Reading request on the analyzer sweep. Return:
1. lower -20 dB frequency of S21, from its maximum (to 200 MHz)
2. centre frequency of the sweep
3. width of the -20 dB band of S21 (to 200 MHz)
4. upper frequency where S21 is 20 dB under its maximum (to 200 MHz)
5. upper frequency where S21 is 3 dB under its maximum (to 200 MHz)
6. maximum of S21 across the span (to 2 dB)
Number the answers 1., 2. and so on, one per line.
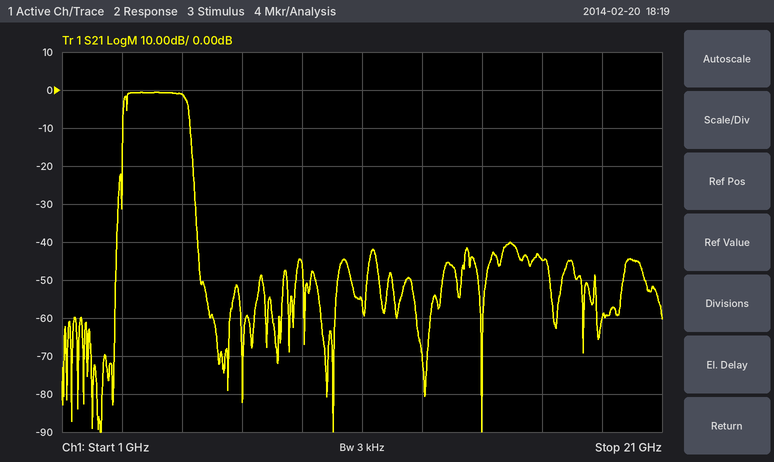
1. 3.0 GHz
2. 11 GHz
3. 2.4 GHz
4. 5.4 GHz
5. 5.2 GHz
6. 0 dB
